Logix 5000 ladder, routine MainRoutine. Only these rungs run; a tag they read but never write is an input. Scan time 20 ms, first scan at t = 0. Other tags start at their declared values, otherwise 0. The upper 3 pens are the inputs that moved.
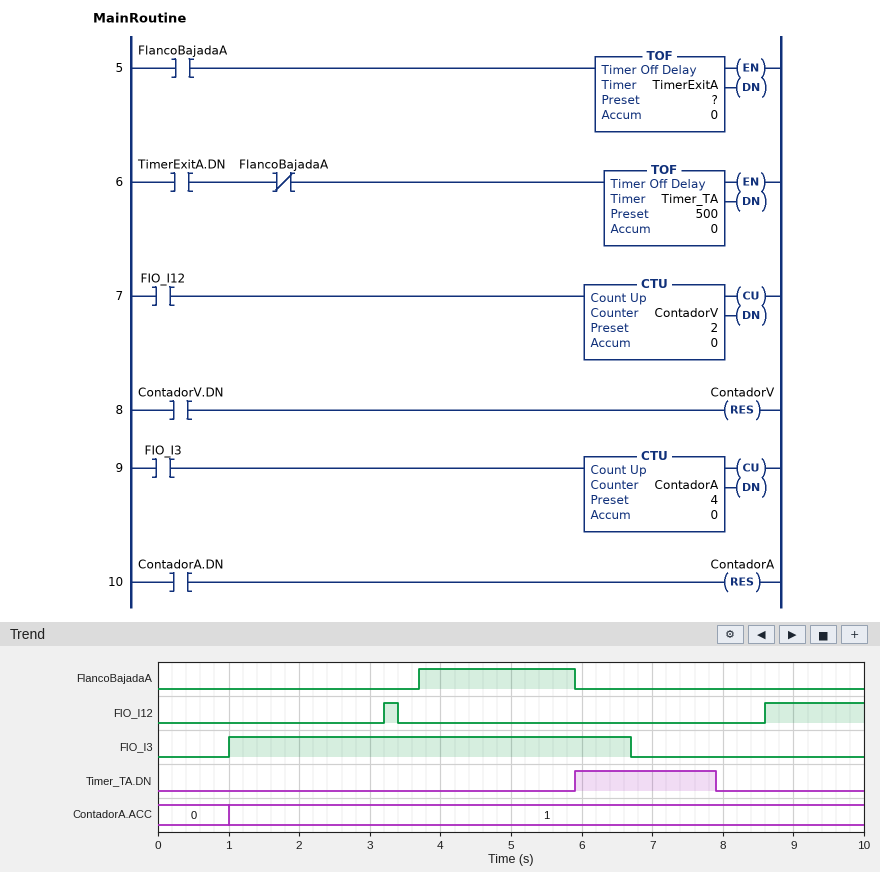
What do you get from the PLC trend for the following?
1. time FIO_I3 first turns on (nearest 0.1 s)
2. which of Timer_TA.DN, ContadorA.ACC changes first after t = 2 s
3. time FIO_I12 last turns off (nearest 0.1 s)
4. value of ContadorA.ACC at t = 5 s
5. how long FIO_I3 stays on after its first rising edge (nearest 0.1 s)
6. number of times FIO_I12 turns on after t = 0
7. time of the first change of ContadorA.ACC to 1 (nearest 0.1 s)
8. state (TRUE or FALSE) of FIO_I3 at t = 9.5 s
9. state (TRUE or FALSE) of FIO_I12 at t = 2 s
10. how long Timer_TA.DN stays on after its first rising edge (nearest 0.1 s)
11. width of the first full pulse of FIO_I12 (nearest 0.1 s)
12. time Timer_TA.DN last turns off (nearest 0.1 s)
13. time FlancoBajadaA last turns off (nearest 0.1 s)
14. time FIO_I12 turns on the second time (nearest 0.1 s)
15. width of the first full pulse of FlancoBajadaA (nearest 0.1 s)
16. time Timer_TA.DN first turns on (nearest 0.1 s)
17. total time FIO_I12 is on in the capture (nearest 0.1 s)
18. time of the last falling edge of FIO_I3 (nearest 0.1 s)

1.0 s
Timer_TA.DN
3.4 s
1
5.7 s
2
1.0 s
FALSE
FALSE
2.0 s
0.2 s
7.9 s
5.9 s
8.6 s
2.2 s
5.9 s
1.6 s
6.7 s
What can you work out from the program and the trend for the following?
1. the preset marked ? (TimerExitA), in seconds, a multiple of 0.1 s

1.5 s
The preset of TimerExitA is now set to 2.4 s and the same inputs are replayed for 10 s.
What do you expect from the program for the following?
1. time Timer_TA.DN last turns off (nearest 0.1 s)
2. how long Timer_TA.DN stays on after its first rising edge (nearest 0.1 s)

8.8 s
2.9 s
